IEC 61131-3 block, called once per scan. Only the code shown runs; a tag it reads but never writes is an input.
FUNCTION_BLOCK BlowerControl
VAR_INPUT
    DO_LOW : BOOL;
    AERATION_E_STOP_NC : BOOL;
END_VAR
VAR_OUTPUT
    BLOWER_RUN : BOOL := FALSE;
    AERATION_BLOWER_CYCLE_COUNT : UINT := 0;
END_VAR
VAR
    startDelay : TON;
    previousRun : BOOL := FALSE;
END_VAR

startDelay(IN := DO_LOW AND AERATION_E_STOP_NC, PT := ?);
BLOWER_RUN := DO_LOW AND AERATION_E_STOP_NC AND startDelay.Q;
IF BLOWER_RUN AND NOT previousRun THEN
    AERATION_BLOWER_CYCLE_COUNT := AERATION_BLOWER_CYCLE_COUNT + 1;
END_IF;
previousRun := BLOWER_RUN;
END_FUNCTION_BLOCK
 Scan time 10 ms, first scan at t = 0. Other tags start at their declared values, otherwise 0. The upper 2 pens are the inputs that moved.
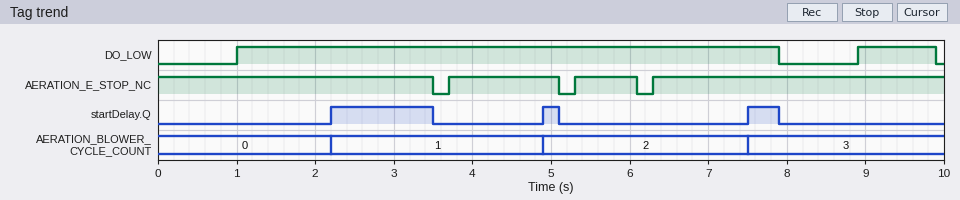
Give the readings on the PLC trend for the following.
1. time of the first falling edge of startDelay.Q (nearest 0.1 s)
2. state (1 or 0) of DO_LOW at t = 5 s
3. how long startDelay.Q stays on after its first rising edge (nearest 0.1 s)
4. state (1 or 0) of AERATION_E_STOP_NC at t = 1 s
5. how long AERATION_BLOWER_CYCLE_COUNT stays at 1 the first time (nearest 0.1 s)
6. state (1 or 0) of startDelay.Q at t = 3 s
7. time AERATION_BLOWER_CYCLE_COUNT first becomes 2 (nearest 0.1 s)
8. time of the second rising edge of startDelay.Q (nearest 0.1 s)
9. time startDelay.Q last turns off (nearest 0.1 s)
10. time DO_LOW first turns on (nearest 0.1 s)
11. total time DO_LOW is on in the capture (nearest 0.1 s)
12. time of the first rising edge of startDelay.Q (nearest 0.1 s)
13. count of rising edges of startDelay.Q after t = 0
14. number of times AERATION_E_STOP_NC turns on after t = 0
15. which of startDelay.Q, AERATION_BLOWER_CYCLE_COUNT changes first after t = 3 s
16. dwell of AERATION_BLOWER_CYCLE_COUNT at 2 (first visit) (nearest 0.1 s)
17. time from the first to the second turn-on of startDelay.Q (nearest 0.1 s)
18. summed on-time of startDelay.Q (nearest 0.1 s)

3.5 s
1
1.3 s
1
2.7 s
1
4.9 s
4.9 s
7.9 s
1.0 s
7.9 s
2.2 s
3
3
startDelay.Q
2.6 s
2.7 s
1.9 s
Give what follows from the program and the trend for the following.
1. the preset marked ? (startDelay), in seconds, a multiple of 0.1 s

1.2 s
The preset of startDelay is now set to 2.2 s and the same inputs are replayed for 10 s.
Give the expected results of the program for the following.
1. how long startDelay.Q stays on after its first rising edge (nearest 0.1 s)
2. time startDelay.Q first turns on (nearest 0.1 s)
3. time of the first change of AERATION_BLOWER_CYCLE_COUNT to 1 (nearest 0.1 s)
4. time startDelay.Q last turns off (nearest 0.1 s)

0.3 s
3.2 s
3.2 s
3.5 s
